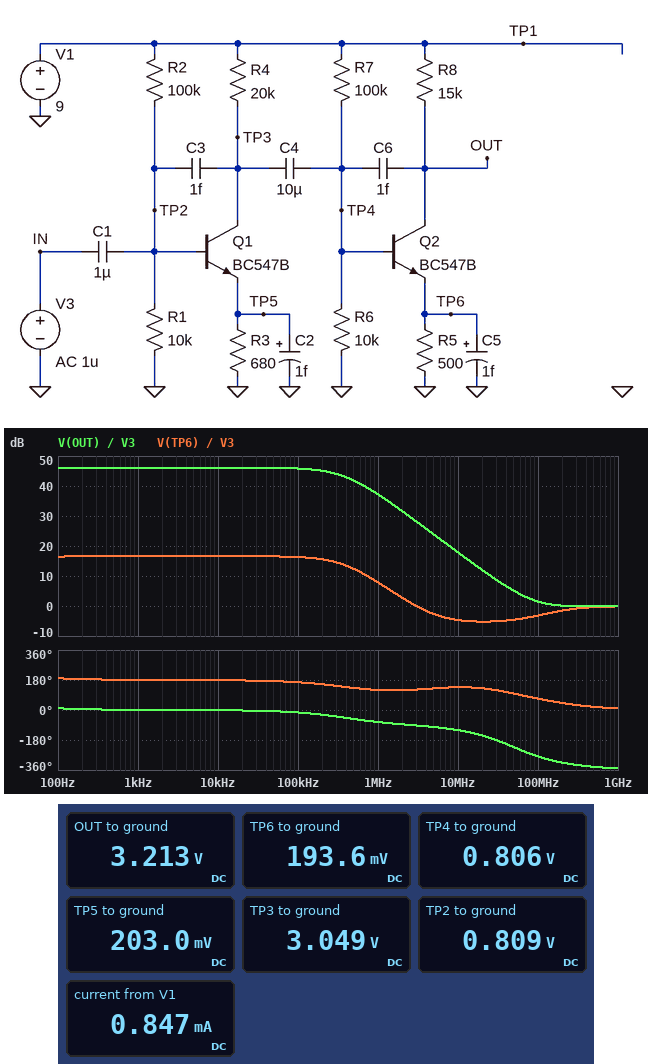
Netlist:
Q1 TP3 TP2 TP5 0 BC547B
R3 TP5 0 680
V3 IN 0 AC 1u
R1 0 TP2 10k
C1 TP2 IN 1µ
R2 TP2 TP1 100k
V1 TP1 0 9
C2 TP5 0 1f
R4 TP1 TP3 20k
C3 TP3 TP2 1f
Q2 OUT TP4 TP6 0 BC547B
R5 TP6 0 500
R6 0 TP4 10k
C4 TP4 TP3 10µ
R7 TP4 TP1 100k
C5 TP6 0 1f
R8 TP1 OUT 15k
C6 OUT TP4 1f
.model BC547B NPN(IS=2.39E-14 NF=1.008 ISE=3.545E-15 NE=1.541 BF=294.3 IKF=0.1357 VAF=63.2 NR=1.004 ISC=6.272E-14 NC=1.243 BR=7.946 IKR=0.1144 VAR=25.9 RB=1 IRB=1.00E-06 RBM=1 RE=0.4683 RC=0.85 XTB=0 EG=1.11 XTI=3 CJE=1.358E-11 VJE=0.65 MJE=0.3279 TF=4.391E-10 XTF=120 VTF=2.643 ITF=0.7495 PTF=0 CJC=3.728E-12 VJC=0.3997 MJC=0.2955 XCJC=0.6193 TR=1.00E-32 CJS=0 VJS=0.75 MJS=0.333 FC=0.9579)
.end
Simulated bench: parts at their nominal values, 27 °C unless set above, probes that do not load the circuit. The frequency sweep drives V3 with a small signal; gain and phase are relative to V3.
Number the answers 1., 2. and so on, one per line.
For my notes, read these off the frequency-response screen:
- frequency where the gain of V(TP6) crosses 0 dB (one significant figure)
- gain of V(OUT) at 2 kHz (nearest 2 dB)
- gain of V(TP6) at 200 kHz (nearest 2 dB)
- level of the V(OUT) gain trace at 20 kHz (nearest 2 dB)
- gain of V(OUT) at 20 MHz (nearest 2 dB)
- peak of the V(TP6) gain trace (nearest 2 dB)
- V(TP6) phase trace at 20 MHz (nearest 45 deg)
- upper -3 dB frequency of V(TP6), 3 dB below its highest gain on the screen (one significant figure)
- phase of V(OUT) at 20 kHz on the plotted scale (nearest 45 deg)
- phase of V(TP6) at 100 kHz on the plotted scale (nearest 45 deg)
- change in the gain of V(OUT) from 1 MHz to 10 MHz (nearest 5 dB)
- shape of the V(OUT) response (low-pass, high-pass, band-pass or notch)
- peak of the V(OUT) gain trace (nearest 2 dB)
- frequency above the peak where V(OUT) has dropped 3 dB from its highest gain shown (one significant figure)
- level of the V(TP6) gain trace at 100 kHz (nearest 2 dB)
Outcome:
1. 3 MHz
2. 46 dB
3. 16 dB
4. 46 dB
5. 12 dB
6. 16 dB
7. 135 deg
8. 400 kHz
9. 0 deg
10. 180 deg
11. -20 dB
12. low-pass
13. 46 dB
14. 400 kHz
15. 16 dB
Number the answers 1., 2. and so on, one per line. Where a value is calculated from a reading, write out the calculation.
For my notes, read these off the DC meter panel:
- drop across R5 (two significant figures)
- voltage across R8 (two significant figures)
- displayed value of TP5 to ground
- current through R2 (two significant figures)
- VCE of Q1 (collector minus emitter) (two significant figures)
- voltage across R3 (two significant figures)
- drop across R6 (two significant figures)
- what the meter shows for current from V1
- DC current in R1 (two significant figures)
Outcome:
1. 193.6 mV = 190 mV
2. 9 V - 3.213 V = 5.8 V
3. 203.0 mV
4. (9 V - 809 mV) / 100 kΩ = 82 µA
5. 3.049 V - 203 mV = 2.8 V
6. 203 mV = 200 mV
7. 806 mV = 810 mV
8. 0.847 mA
9. (809 mV) / 10 kΩ = 81 µA
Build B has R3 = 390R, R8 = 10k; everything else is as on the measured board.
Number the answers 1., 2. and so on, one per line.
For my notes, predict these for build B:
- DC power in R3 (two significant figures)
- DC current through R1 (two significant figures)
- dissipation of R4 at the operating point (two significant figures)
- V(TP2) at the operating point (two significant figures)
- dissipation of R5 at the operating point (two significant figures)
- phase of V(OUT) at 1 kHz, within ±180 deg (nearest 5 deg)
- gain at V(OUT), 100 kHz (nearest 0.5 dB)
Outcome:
1. 75 µW
2. 79 µA
3. 3.8 mW
4. 790 mV
5. 76 µW
6. 5 deg
7. 42.5 dB
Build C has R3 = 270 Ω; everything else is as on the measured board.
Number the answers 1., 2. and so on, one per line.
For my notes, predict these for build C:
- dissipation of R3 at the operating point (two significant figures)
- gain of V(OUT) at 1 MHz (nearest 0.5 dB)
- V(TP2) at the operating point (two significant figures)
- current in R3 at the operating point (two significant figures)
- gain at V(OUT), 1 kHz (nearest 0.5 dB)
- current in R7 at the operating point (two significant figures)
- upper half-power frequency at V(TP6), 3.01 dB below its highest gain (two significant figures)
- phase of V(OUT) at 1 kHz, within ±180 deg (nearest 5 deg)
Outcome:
1. 54 µW
2. 36.5 dB
3. 740 mV
4. 450 µA
5. 40.0 dB
6. 82 µA
7. 950 kHz
8. 10 deg
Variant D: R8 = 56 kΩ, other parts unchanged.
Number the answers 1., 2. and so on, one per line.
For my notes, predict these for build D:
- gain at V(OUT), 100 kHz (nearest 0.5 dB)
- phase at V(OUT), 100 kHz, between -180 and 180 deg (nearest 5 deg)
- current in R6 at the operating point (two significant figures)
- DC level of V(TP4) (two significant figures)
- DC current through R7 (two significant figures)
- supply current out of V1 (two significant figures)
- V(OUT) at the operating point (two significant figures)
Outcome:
1. -2.0 dB
2. -5 deg
3. 69 µA
4. 690 mV
5. 83 µA
6. 620 µA
7. 120 mV
